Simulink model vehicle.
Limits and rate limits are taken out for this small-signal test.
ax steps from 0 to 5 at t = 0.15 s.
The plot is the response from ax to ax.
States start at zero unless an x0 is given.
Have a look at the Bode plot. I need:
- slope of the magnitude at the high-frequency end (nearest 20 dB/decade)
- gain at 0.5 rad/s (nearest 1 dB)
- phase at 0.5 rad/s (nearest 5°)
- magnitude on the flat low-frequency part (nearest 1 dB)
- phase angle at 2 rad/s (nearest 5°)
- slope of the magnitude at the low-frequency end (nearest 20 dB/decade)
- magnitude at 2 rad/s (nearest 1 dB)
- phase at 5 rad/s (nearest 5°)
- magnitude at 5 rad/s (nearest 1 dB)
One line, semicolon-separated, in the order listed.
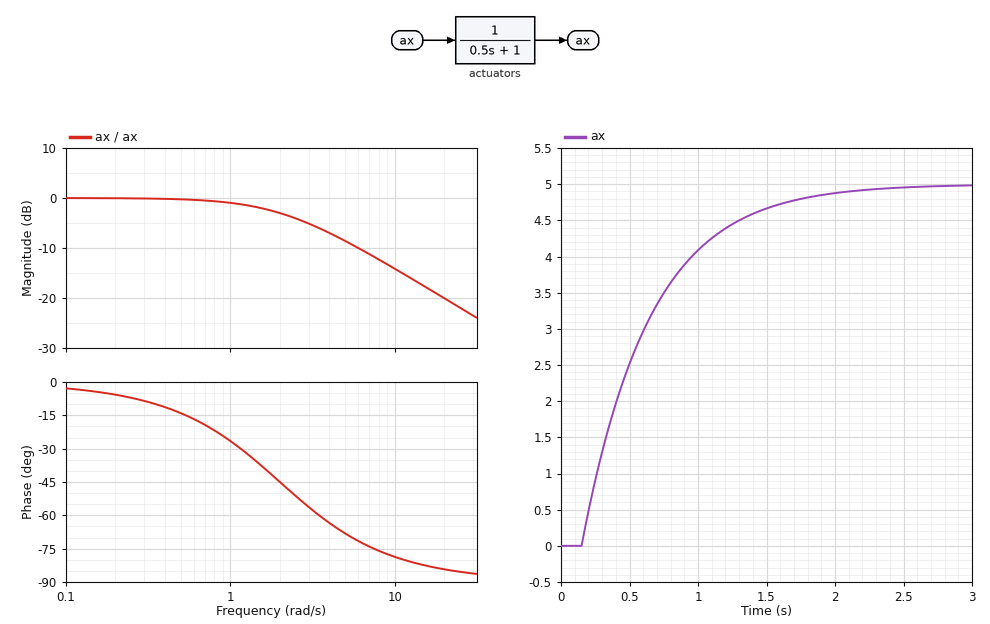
-20 dB/decade; 0 dB; -15°; 0 dB; -45°; 0 dB/decade; -3 dB; -70°; -9 dB
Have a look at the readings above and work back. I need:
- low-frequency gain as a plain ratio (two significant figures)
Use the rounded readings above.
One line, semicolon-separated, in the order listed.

1.0
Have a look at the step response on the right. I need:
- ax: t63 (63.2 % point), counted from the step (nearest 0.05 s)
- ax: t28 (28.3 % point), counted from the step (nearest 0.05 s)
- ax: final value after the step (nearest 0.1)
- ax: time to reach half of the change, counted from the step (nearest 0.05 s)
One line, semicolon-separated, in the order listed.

0.50 s; 0.15 s; 5.0; 0.35 s
